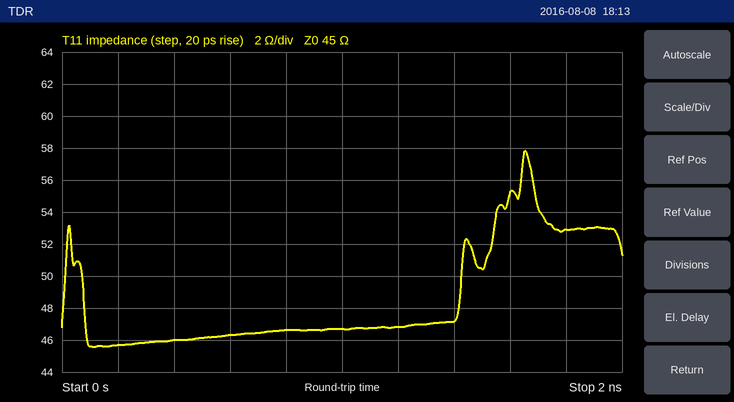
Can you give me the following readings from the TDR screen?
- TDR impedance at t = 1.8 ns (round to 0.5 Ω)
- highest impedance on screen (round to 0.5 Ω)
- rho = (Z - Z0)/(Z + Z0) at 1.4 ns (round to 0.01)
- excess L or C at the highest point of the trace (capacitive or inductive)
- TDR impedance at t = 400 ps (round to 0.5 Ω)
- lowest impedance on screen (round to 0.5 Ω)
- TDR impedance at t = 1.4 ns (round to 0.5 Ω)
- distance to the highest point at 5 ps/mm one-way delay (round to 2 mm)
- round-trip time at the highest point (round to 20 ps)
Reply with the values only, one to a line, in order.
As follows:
53.0 Ω
58.0 Ω
+0.02
inductive
46.0 Ω
45.5 Ω
47.0 Ω
166 mm
1.66 ns
